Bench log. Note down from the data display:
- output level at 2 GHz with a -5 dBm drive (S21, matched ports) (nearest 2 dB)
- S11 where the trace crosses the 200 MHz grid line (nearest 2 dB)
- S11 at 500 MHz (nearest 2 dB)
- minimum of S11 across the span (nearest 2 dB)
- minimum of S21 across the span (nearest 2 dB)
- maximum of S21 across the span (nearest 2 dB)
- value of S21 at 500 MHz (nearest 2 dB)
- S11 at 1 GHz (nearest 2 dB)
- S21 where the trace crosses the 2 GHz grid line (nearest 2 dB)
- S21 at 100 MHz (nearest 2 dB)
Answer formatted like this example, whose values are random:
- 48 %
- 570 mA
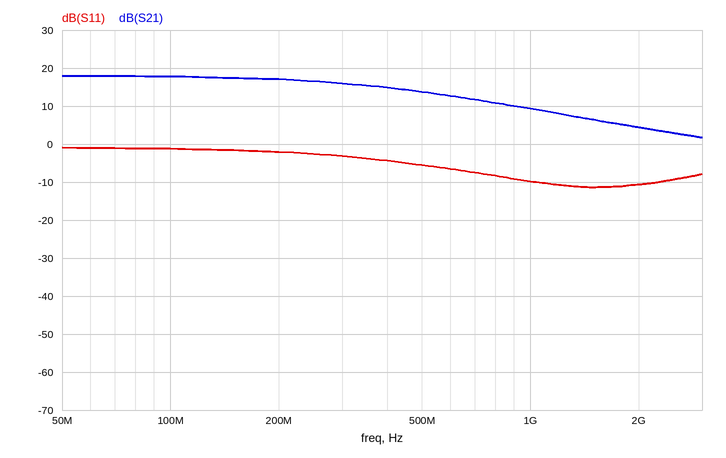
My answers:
- 0 dBm
- -2 dB
- -6 dB
- -12 dB
- 2 dB
- 18 dB
- 14 dB
- -10 dB
- 4 dB
- 18 dB
